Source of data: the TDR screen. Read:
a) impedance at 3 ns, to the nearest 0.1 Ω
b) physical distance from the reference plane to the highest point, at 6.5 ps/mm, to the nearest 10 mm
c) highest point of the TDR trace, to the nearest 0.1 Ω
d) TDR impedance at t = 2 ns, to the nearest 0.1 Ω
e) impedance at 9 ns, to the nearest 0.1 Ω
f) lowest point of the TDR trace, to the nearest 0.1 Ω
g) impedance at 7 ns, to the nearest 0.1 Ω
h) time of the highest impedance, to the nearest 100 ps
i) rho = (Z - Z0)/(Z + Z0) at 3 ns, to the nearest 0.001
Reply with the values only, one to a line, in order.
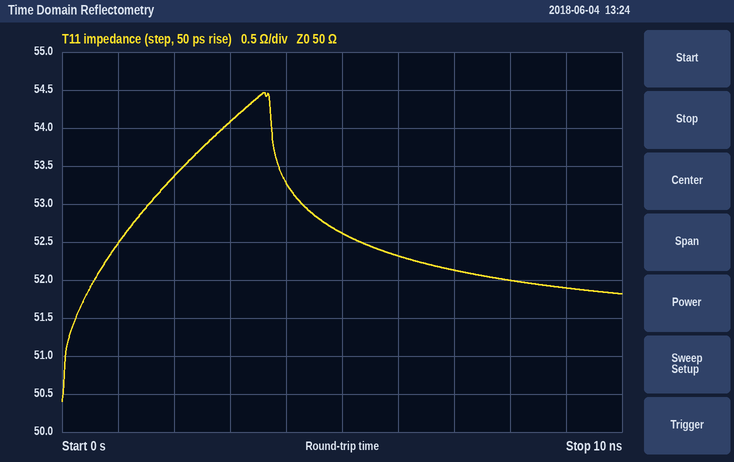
54.1 Ω
280 mm
54.5 Ω
53.4 Ω
51.9 Ω
50.4 Ω
52.1 Ω
3.6 ns
+0.039
